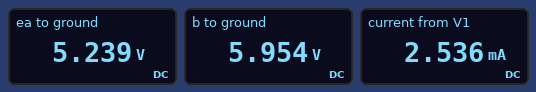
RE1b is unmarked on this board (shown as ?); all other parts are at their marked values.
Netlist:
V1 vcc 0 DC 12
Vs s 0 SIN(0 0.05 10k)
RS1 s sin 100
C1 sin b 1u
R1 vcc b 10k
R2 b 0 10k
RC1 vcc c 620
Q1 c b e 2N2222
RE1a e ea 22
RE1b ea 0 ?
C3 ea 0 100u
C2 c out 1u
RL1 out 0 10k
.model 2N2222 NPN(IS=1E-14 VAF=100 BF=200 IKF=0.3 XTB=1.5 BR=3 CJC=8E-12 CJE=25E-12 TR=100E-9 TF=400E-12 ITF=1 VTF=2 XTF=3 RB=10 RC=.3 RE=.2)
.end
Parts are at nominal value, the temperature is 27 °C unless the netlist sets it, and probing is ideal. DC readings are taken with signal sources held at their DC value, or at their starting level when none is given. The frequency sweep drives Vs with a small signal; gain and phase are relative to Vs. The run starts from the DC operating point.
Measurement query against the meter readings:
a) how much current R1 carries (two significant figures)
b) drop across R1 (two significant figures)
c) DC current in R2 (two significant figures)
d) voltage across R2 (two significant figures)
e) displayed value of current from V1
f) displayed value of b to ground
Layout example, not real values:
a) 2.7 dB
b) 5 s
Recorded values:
a) 600 µA
b) 6.0 V
c) 600 µA
d) 6.0 V
e) 2.536 mA
f) 5.954 V
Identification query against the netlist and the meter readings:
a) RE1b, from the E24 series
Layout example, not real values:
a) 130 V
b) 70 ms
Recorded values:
a) 2.7 kΩ
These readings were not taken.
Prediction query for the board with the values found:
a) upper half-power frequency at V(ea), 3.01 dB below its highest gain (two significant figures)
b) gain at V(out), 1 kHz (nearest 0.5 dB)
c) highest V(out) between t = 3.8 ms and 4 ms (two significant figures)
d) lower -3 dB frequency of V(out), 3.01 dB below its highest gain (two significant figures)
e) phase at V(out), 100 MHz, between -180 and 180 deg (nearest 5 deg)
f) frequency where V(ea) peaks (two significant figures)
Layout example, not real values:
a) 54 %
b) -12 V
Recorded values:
a) 110 Hz
b) 24.0 dB
c) 700 mV
d) 85 Hz
e) 70 deg
f) 37 Hz
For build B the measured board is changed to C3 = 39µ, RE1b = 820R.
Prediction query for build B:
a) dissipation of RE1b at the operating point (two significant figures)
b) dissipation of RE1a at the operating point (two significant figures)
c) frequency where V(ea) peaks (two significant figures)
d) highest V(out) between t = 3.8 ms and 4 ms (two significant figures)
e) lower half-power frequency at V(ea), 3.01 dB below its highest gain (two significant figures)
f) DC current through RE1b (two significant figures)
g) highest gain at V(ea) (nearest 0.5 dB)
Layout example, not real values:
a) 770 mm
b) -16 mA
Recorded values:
a) 31 mW
b) 820 µW
c) 71 Hz
d) 1.0 V
e) 21 Hz
f) 6.1 mA
g) -3.5 dB
